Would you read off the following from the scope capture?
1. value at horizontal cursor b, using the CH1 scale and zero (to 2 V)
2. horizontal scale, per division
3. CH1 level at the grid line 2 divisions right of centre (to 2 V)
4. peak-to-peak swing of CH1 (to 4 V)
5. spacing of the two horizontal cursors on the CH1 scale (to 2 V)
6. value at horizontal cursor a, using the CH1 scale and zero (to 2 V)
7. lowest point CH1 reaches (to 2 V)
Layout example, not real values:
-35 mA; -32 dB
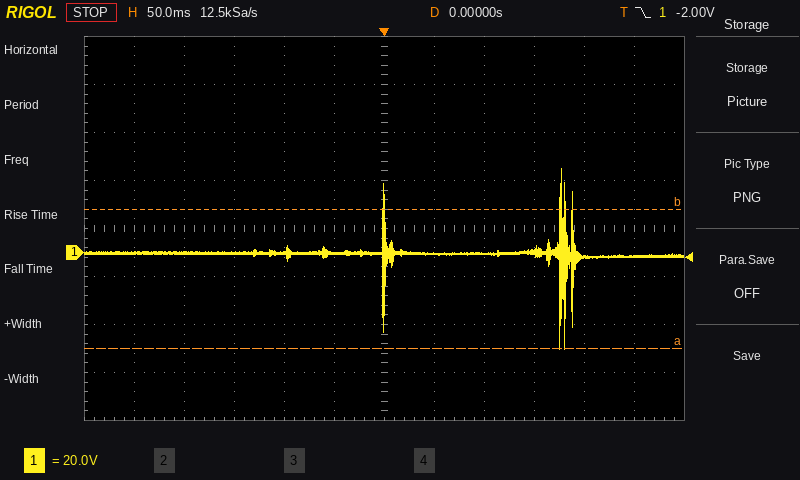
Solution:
18 V; 50 ms; 0 V; 76 V; 58 V; -40 V; -40 V
